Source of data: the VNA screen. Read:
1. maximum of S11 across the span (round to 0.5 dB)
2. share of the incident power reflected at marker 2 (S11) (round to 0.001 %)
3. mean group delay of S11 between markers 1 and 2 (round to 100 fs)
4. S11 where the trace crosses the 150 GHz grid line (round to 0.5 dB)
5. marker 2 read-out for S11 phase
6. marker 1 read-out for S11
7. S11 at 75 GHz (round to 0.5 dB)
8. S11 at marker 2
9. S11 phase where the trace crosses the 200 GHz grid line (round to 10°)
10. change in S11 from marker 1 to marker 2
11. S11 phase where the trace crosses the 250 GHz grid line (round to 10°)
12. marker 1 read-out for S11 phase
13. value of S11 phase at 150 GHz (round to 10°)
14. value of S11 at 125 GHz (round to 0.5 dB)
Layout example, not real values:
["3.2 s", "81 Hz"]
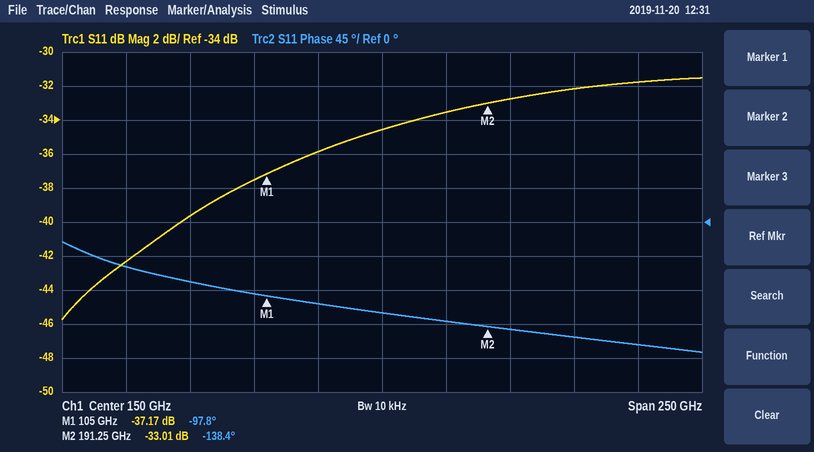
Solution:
["-31.5 dB", "0.050 %", "1.3 ps", "-34.5 dB", "-138.4°", "-37.17 dB", "-39.5 dB", "-33.01 dB", "-140°", "4.16 dB", "-160°", "-97.8°", "-120°", "-36.0 dB"]
